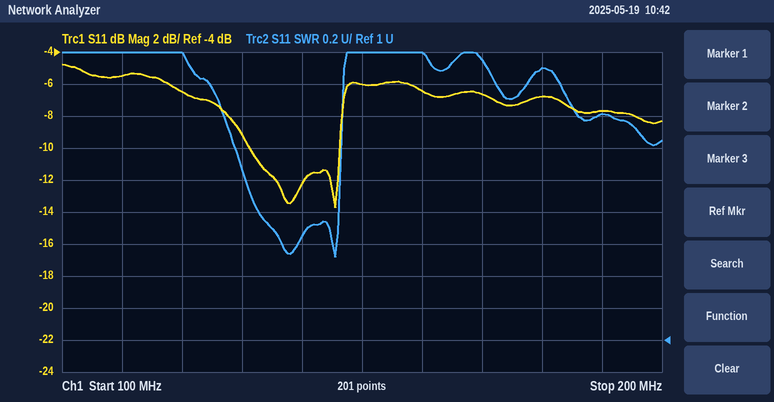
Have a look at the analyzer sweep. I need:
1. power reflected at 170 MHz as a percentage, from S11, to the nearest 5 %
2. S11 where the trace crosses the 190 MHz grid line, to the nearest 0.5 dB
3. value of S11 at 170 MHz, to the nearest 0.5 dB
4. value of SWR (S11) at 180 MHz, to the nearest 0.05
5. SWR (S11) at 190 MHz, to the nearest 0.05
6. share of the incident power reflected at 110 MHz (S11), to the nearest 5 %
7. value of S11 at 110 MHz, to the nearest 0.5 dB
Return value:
20 %
-7.5 dB
-6.5 dB
2.70
2.40
30 %
-5.5 dB
